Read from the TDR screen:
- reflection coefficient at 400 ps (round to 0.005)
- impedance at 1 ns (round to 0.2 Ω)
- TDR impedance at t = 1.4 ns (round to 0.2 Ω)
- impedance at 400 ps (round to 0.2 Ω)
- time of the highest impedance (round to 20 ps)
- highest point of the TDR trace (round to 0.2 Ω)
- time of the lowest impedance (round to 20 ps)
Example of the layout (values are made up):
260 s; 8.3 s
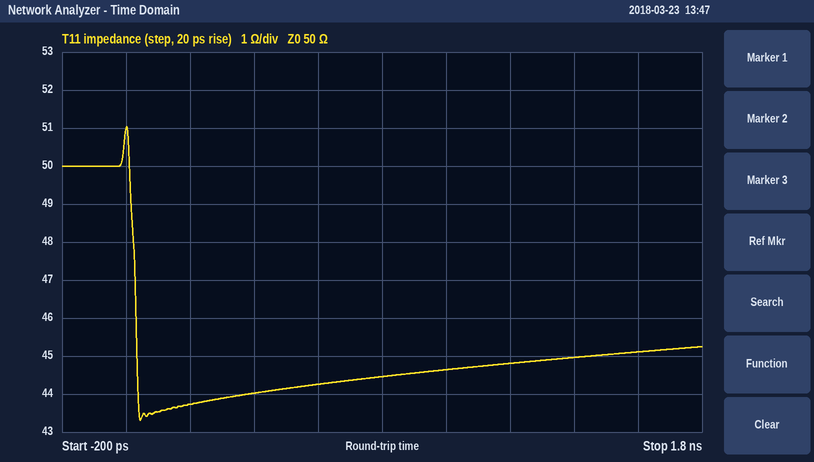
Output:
-0.065; 44.6 Ω; 45.0 Ω; 44.0 Ω; 0 ps; 51.0 Ω; 40 ps
